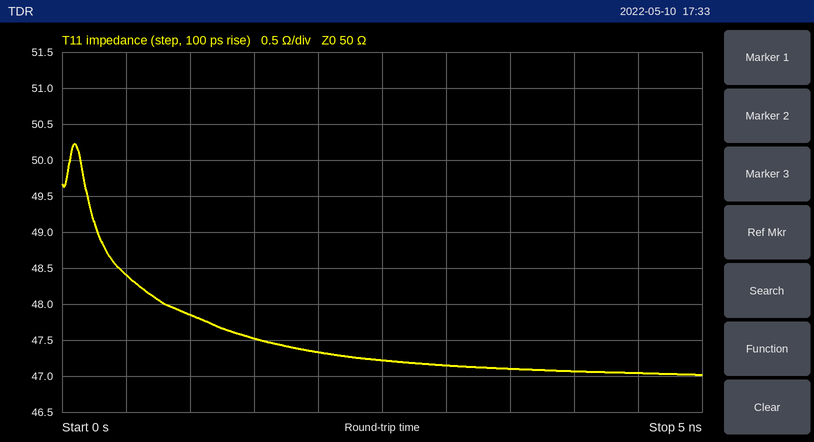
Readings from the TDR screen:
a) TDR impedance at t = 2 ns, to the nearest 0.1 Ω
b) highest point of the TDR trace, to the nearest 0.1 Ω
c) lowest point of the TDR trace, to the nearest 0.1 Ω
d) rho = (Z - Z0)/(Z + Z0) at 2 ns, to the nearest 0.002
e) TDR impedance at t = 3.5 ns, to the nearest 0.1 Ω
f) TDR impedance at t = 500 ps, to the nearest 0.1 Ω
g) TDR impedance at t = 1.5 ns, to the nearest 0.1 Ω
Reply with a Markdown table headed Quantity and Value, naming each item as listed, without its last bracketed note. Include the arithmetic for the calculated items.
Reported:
| Quantity | Value |
|---|---|
| TDR impedance at t = 2 ns, to the nearest 0.1 Ω | 47.3 Ω |
| highest point of the TDR trace, to the nearest 0.1 Ω | 50.2 Ω |
| lowest point of the TDR trace, to the nearest 0.1 Ω | 47.0 Ω |
| rho = (Z - Z0)/(Z + Z0) at 2 ns, to the nearest 0.002 | (47.3 − 50)/(47.3 + 50) ≈ -0.028 |
| TDR impedance at t = 3.5 ns, to the nearest 0.1 Ω | 47.1 Ω |
| TDR impedance at t = 500 ps, to the nearest 0.1 Ω | 48.4 Ω |
| TDR impedance at t = 1.5 ns, to the nearest 0.1 Ω | 47.5 Ω |
